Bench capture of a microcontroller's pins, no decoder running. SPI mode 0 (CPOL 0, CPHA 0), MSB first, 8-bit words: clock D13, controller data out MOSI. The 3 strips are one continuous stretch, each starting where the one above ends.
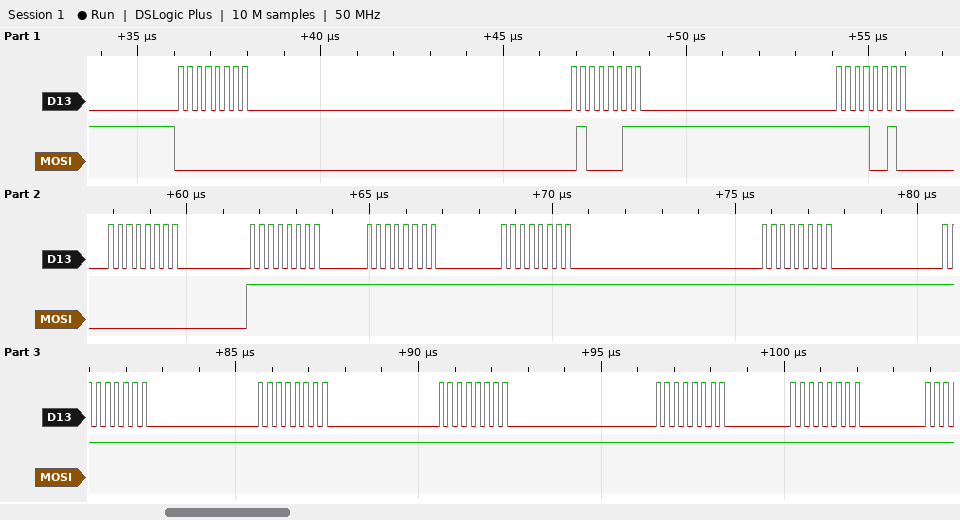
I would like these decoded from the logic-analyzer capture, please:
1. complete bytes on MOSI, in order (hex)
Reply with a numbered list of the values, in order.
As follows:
1. 00 43 F2 00 FF FF FF FF FF FF FF FF FF
